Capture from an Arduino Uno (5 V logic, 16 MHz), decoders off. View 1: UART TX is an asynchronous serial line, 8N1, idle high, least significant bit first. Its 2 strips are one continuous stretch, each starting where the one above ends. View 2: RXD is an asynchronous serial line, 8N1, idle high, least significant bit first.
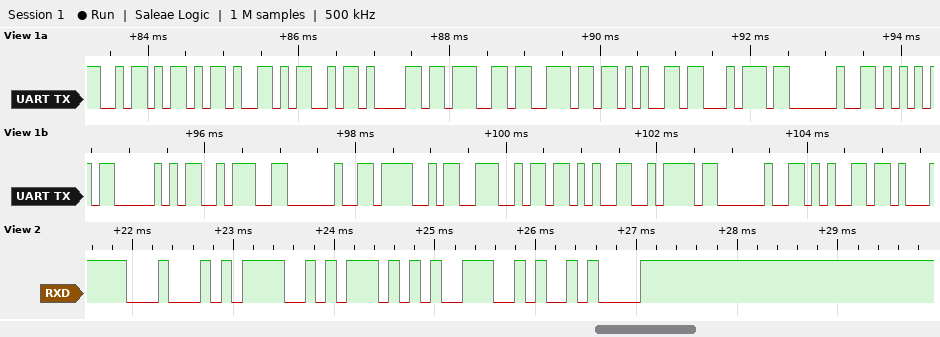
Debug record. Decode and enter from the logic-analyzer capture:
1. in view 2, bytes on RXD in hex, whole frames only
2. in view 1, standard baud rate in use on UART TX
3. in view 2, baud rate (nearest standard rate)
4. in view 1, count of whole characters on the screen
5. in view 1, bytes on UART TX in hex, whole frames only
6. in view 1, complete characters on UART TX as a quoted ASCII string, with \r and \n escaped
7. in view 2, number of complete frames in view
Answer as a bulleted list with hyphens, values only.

- 44 4F 57 4E 0A
- 9600 baud
- 9600 baud
- 19
- 0x5A 0x2D 0x4D 0x61 0x67 0x6E 0x65 0x74 0x20 0x55 0x50 0x3A 0x20 0x4F 0x4E 0x2B 0x7A 0x20 0x65
- "Z-Magnet UP: ON+z e"
- 5
